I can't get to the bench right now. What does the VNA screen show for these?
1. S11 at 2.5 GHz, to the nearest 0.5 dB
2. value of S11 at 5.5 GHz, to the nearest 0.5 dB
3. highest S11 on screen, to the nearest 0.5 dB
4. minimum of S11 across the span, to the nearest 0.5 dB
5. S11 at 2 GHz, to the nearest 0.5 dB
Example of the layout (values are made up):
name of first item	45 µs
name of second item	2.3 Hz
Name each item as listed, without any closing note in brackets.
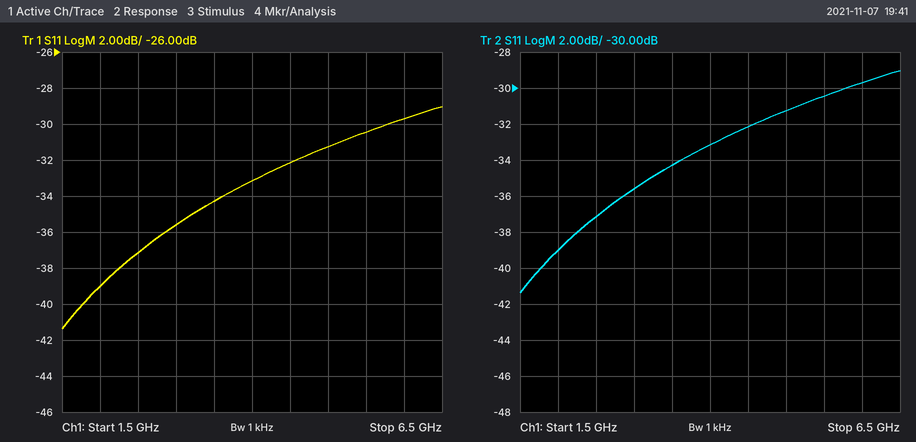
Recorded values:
S11 at 2.5 GHz, to the nearest 0.5 dB	-37.0 dB
value of S11 at 5.5 GHz, to the nearest 0.5 dB	-30.5 dB
highest S11 on screen, to the nearest 0.5 dB	-29.0 dB
minimum of S11 across the span, to the nearest 0.5 dB	-41.5 dB
S11 at 2 GHz, to the nearest 0.5 dB	-39.0 dB
